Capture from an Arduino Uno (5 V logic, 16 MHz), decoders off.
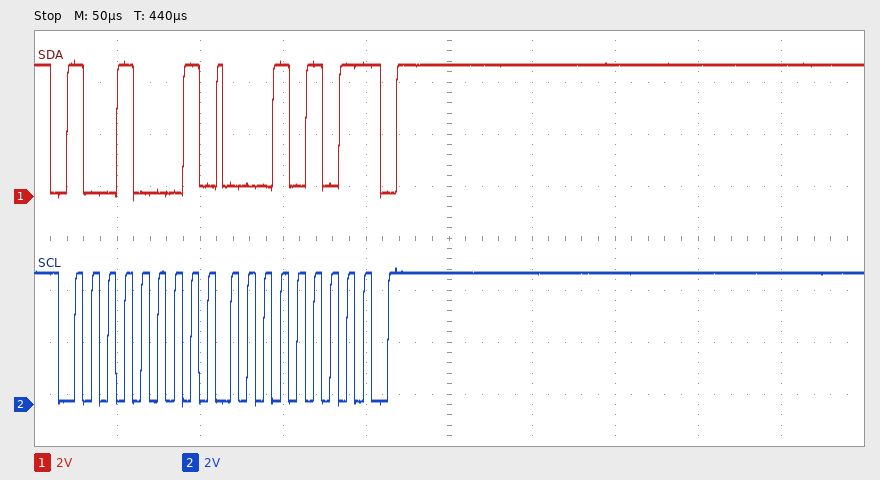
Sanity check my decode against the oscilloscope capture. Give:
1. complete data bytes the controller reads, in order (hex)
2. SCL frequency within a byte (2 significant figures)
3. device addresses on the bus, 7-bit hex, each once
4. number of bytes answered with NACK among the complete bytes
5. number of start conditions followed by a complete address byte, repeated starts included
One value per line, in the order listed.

15
100 kHz
0x48
1
1
